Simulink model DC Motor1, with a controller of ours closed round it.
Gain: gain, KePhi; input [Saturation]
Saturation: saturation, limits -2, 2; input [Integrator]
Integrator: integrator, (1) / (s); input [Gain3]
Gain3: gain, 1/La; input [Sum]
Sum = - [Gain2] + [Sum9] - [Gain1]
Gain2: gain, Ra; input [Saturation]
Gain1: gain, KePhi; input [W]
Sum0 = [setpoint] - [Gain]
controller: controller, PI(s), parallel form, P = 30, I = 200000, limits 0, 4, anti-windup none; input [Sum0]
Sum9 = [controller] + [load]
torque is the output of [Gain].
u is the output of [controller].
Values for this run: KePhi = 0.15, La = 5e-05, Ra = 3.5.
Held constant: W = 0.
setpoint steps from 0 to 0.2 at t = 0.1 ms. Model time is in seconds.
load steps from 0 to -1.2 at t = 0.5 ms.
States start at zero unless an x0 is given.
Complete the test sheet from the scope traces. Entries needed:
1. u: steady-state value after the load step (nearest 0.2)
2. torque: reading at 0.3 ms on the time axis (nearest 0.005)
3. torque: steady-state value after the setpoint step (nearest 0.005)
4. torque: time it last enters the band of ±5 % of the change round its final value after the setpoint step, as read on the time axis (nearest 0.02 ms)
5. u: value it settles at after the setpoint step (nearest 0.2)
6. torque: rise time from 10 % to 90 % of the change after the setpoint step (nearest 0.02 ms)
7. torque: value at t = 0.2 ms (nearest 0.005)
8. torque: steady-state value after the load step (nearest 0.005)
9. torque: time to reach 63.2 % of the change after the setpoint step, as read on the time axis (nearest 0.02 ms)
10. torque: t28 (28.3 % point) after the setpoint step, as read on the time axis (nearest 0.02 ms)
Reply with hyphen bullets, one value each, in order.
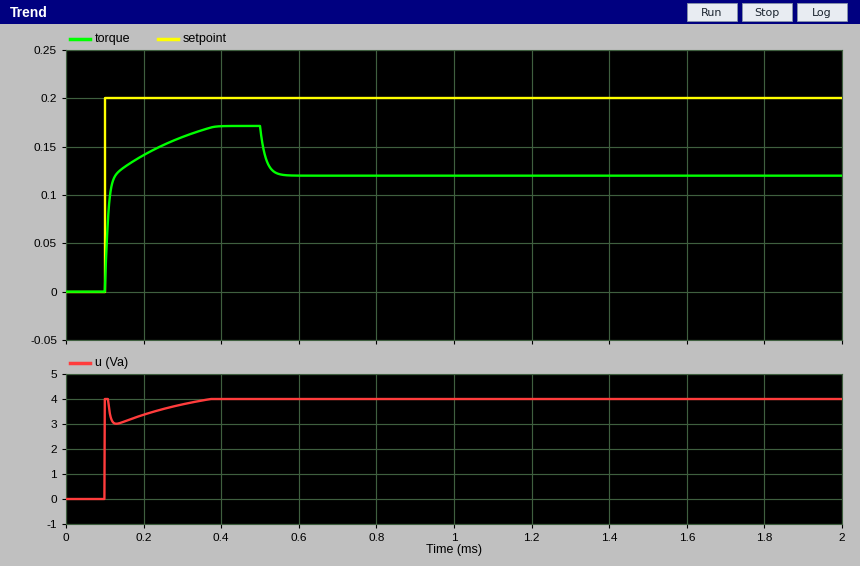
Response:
- 4.0
- 0.160
- 0.170
- 0.32 ms
- 4.0
- 0.16 ms
- 0.140
- 0.120
- 0.12 ms
- 0.10 ms
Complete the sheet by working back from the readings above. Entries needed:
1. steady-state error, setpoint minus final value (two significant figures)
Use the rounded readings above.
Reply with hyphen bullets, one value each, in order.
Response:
- 0.030
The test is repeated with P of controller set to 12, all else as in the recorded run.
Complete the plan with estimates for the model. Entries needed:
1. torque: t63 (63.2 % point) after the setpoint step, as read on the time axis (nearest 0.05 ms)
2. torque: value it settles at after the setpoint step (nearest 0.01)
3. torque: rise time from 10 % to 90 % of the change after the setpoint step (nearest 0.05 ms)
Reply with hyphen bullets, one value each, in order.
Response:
- 0.15 ms
- 0.17
- 0.20 ms
